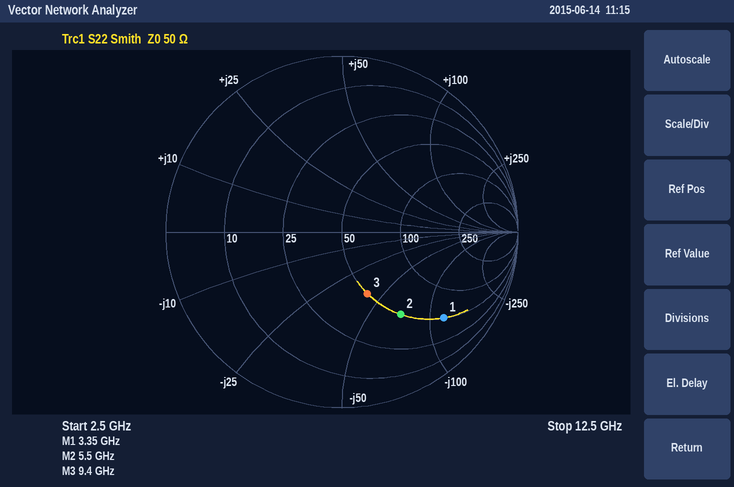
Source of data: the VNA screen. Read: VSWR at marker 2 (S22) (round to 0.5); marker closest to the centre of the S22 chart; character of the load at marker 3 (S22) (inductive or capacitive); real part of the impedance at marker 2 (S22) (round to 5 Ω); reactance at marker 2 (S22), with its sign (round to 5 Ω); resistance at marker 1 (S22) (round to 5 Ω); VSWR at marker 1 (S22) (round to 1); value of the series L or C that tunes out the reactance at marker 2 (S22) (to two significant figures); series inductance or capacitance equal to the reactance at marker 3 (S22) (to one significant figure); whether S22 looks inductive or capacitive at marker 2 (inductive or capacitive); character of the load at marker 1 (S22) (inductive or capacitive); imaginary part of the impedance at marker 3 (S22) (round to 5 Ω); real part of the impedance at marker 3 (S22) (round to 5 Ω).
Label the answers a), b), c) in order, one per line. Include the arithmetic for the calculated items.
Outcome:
a) 3.5
b) marker 3
c) capacitive
d) 50 Ω
e) -70 Ω
f) 50 Ω
g) 7
h) L = 70 Ω/(2π × 5.5 GHz) ≈ 2.0 nH
i) C = 1/(2π × 9.4 GHz × 40 Ω) ≈ 423 fF, so 400 fF to one significant figure
j) capacitive
k) capacitive
l) -40 Ω
m) 50 Ω
